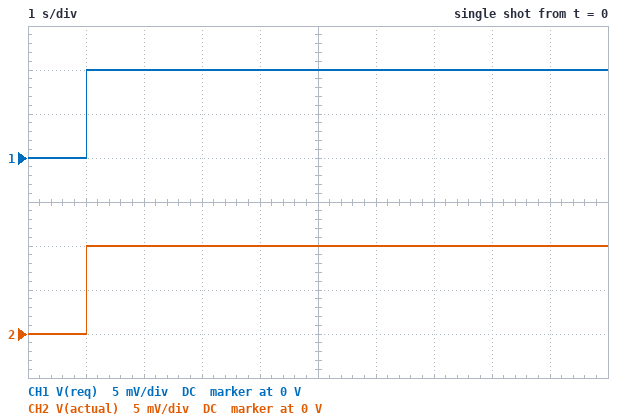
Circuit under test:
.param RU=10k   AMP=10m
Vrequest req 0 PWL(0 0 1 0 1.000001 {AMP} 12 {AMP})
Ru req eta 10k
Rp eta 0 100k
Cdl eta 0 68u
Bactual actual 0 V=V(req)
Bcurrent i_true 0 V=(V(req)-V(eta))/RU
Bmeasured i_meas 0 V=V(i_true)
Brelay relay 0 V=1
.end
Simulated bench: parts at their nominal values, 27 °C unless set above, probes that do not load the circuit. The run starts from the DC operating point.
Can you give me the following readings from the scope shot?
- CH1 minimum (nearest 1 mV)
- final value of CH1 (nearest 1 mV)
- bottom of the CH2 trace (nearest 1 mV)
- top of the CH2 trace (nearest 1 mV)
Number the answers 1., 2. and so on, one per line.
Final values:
1. 0 V
2. 10 mV
3. 0 V
4. 10 mV
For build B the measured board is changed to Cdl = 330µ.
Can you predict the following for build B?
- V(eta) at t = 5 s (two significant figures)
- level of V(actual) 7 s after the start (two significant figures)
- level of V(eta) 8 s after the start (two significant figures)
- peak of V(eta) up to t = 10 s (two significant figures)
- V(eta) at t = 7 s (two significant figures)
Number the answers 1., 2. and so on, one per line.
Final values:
1. 6.7 mV
2. 10 mV
3. 8.2 mV
4. 8.6 mV
5. 7.9 mV
